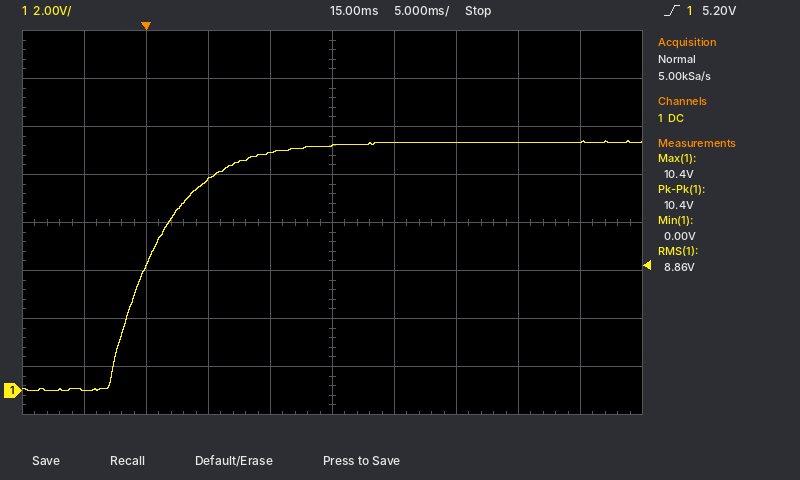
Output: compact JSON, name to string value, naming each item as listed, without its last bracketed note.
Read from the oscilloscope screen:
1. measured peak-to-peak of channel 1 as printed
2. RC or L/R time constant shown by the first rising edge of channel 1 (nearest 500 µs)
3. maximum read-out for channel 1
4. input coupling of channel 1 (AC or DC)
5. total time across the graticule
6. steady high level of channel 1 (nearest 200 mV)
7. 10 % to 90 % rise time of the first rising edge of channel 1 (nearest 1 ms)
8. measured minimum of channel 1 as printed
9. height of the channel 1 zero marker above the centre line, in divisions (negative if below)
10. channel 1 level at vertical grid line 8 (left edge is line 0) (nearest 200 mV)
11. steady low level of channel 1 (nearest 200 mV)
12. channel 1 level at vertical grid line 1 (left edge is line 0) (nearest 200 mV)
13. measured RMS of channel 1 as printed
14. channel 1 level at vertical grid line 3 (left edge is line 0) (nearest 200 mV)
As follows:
{"measured peak-to-peak of channel 1 as printed": "10.4 V", "RC or L/R time constant shown by the first rising edge of channel 1": "4.0 ms", "maximum read-out for channel 1": "10.4 V", "input coupling of channel 1": "DC", "total time across the graticule": "50 ms", "steady high level of channel 1": "10.4 V", "10 % to 90 % rise time of the first rising edge of channel 1": "9 ms", "measured minimum of channel 1 as printed": "0.00 V", "height of the channel 1 zero marker above the centre line, in divisions": "-3.5 div", "channel 1 level at vertical grid line 8 (left edge is line 0)": "10.4 V", "steady low level of channel 1": "0.0 V", "channel 1 level at vertical grid line 1 (left edge is line 0)": "0.0 V", "measured RMS of channel 1 as printed": "8.86 V", "channel 1 level at vertical grid line 3 (left edge is line 0)": "8.8 V"}
